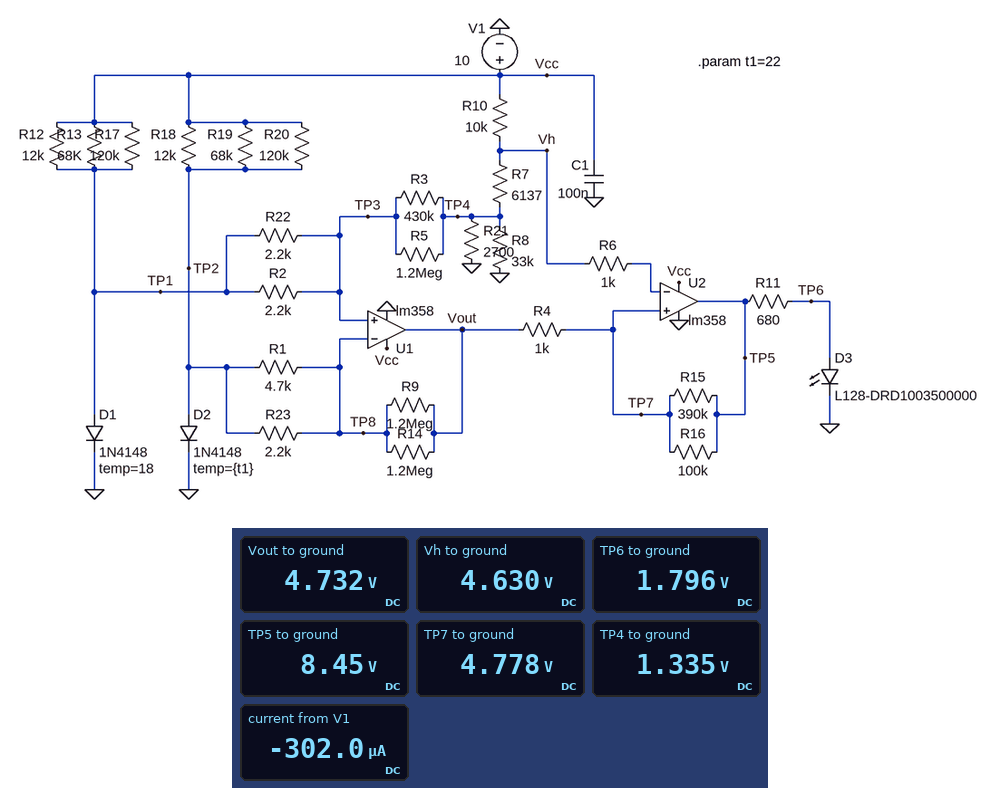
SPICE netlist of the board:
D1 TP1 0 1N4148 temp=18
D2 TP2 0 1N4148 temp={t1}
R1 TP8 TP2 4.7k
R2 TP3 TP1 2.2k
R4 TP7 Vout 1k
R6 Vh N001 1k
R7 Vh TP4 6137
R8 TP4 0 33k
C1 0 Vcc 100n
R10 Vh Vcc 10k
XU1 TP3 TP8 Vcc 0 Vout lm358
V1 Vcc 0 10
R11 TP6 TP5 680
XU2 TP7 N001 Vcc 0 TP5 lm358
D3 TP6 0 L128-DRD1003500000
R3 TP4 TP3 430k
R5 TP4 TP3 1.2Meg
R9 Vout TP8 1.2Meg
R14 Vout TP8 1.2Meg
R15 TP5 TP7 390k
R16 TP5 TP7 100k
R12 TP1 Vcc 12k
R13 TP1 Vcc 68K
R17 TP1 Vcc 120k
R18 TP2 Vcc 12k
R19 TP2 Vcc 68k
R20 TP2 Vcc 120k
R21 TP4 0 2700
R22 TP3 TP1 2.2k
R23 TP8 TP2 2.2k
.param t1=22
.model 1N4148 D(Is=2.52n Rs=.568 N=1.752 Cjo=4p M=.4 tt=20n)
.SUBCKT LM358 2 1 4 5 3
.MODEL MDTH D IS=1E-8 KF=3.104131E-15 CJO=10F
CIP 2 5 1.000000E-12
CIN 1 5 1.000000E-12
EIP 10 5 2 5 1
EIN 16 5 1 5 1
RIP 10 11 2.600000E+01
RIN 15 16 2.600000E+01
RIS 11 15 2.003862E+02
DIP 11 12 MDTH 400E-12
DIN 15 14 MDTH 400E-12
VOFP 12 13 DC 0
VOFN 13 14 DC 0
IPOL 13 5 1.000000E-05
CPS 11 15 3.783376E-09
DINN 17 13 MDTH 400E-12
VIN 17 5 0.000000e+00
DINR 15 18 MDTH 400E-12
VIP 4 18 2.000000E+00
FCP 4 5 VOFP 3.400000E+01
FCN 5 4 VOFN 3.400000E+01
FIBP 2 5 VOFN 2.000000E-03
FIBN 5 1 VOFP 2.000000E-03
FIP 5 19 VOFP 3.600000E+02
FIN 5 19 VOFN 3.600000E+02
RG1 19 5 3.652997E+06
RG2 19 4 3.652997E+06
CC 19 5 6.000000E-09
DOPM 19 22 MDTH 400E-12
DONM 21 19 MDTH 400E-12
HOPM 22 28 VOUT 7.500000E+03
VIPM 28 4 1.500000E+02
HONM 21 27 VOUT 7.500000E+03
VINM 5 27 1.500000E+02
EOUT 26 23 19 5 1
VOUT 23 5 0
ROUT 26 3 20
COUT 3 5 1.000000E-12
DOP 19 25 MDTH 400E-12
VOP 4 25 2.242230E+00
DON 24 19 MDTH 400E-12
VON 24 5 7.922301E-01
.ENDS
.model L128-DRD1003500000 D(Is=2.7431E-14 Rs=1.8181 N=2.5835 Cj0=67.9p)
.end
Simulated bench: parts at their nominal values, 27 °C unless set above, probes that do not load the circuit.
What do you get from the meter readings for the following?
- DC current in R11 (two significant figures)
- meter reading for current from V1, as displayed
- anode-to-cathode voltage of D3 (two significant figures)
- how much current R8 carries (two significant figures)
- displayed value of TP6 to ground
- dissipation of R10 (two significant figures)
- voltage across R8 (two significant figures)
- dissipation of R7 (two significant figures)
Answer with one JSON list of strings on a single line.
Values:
["9.8 mA", "-302.0 µA", "1.8 V", "40 µA", "1.796 V", "2.9 mW", "1.3 V", "1.8 mW"]
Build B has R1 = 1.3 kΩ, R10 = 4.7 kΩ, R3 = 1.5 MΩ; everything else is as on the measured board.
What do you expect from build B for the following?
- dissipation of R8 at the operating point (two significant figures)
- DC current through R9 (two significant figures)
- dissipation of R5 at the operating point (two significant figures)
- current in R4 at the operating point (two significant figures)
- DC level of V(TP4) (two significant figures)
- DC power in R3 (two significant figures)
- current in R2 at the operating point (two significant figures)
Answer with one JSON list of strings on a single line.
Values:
["110 µW", "5.9 µA", "1.3 µW", "9.9 µA", "1.9 V", "1.1 µW", "950 nA"]
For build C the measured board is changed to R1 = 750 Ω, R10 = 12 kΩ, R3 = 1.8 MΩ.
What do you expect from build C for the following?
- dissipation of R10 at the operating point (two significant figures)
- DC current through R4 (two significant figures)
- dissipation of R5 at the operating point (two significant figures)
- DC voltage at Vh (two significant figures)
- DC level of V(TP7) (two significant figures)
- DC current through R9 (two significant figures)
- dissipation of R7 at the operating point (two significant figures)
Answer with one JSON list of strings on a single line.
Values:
["2.8 mW", "1.1 µA", "300 nW", "4.2 V", "8.5 V", "6.6 µA", "1.4 mW"]
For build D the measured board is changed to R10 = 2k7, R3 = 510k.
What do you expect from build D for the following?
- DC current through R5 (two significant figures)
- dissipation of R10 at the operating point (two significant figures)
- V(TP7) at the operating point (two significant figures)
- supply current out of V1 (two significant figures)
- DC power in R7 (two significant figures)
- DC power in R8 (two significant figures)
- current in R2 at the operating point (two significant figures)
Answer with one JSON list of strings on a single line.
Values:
["1.3 µA", "2.1 mW", "5.6 V", "3.6 mA", "4.8 mW", "150 µW", "2.2 µA"]
